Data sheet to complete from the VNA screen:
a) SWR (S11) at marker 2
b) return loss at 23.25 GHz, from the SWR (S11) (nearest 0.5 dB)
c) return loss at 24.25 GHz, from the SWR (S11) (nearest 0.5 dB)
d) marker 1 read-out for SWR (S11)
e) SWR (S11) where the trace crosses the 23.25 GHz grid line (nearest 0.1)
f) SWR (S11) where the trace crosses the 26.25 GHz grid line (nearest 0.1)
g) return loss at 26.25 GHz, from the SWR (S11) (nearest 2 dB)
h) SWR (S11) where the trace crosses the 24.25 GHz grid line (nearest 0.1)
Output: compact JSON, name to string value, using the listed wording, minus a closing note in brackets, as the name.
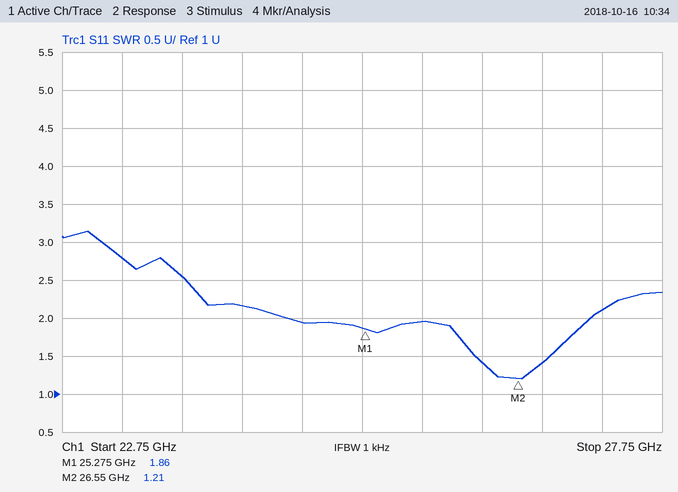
{"SWR (S11) at marker 2": "1.21", "return loss at 23.25 GHz, from the SWR (S11)": "6.5 dB", "return loss at 24.25 GHz, from the SWR (S11)": "8.5 dB", "marker 1 read-out for SWR": "1.86", "SWR (S11) where the trace crosses the 23.25 GHz grid line": "2.8", "SWR (S11) where the trace crosses the 26.25 GHz grid line": "1.4", "return loss at 26.25 GHz, from the SWR (S11)": "16 dB", "SWR (S11) where the trace crosses the 24.25 GHz grid line": "2.2"}
